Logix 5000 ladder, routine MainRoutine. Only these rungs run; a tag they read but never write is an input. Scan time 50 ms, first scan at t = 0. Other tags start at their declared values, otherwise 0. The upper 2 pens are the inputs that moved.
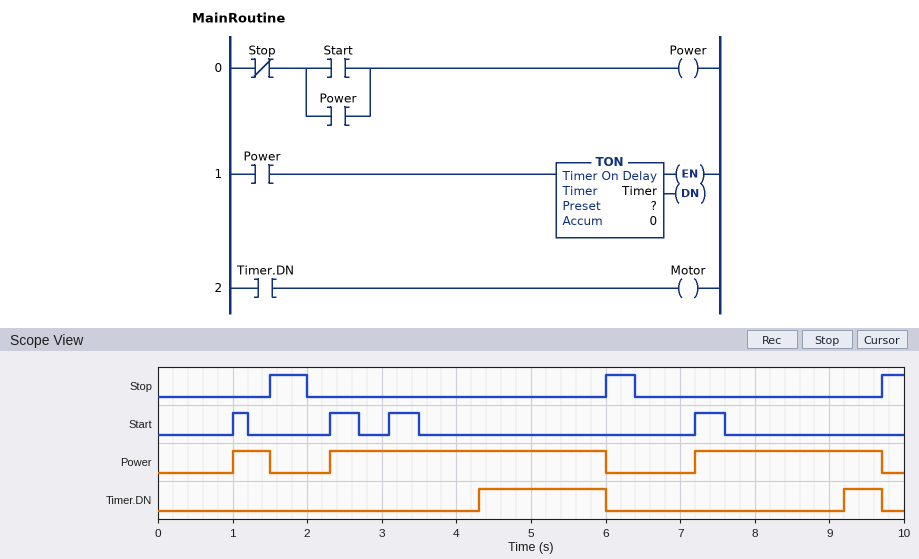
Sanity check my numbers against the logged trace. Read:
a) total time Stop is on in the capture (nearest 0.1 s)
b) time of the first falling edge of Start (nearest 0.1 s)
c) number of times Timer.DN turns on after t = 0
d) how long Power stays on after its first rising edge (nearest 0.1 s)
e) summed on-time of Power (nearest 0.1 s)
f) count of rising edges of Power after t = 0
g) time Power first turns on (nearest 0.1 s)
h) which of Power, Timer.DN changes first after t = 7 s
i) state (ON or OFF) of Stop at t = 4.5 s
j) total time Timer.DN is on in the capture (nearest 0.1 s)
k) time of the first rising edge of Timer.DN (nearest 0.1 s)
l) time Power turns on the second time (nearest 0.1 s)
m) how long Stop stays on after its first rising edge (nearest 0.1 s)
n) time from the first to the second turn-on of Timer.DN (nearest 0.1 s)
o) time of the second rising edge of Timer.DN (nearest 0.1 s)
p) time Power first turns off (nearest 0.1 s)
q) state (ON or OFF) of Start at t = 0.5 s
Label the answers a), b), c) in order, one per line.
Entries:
a) 1.2 s
b) 1.2 s
c) 2
d) 0.5 s
e) 6.7 s
f) 3
g) 1.0 s
h) Power
i) OFF
j) 2.2 s
k) 4.3 s
l) 2.3 s
m) 0.5 s
n) 4.9 s
o) 9.2 s
p) 1.5 s
q) OFF
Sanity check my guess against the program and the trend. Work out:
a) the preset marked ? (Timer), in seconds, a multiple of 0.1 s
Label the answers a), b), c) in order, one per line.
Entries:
a) 2.0 s
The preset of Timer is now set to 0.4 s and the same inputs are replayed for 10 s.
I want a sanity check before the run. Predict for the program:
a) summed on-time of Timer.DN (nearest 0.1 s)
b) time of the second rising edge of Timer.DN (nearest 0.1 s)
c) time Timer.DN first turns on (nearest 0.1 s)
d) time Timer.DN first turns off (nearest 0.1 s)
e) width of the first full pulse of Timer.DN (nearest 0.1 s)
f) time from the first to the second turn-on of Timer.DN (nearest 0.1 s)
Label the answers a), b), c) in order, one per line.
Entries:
a) 5.5 s
b) 2.7 s
c) 1.4 s
d) 1.5 s
e) 0.1 s
f) 1.3 s
